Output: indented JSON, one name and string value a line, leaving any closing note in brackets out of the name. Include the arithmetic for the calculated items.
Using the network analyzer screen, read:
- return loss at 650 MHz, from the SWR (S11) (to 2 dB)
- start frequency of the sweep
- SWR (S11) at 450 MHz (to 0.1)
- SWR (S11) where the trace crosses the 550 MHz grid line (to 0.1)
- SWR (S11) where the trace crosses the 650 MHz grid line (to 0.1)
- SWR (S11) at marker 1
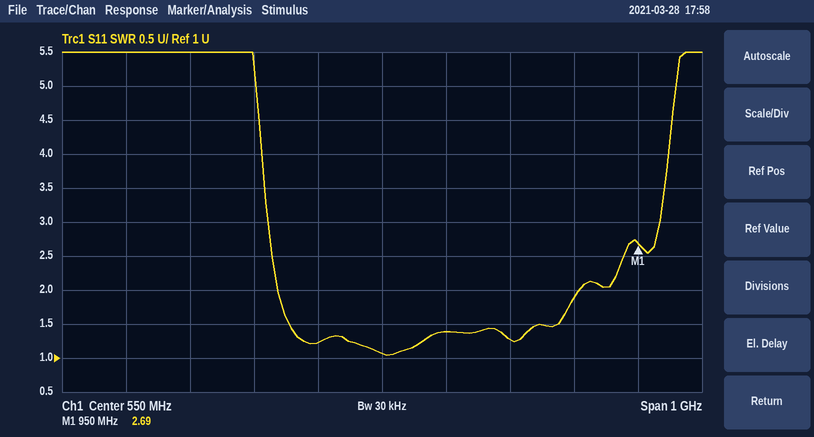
{
  "return loss at 650 MHz, from the SWR (S11)": "−20 log10((1.4 − 1)/(1.4 + 1)) ≈ 16 dB",
  "start frequency of the sweep": "50 MHz",
  "SWR (S11) at 450 MHz": "1.2",
  "SWR (S11) where the trace crosses the 550 MHz grid line": "1.1",
  "SWR (S11) where the trace crosses the 650 MHz grid line": "1.4",
  "SWR (S11) at marker 1": "2.69"
}
